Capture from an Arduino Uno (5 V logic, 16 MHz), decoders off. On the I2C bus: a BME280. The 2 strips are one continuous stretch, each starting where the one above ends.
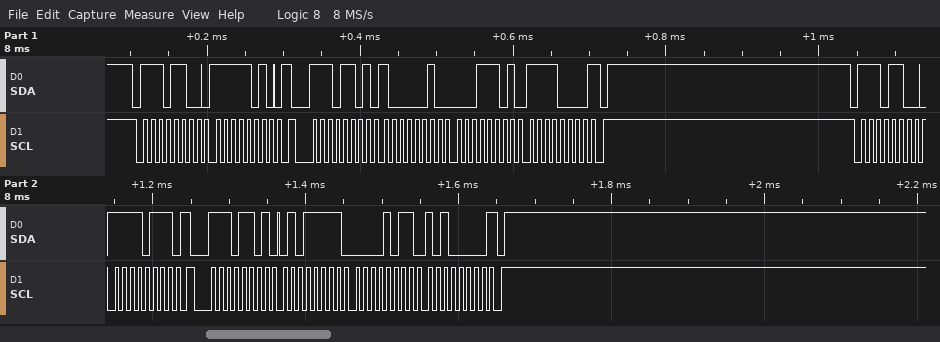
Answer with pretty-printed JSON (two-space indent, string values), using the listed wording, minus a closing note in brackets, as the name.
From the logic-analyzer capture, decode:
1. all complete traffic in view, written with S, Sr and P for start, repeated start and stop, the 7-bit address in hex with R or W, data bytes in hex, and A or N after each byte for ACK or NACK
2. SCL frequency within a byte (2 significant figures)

{
  "all complete traffic in view, written with S, Sr and P for start, repeated start and stop, the 7-bit address in hex with R or W, data bytes in hex, and A or N after each byte for ACK or NACK": "S 76W A FA A Sr 76R A 82 A 1D A F0 N P S 76W A F7 A Sr 76R A 5F A 0B A A0 N P",
  "SCL frequency within a byte": "100 kHz"
}
